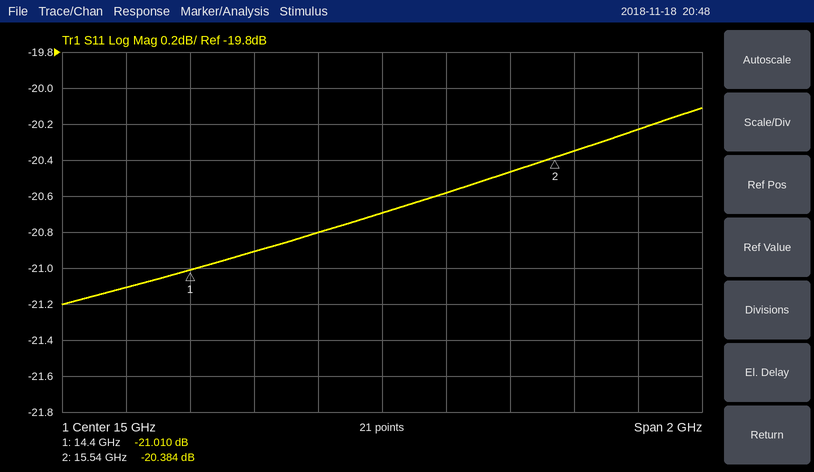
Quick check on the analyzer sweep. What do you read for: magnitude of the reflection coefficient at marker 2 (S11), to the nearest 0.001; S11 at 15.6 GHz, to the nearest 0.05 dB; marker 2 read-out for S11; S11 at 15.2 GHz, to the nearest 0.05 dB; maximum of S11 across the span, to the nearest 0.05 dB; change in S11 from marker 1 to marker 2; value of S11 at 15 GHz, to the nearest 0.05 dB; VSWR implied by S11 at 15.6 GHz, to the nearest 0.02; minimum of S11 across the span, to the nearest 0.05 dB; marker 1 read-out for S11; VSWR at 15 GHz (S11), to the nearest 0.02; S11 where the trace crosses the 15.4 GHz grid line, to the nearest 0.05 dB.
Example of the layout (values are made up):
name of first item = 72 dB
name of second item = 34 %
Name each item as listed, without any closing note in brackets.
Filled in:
magnitude of the reflection coefficient at marker 2 (S11), to the nearest 0.001 = 0.096
S11 at 15.6 GHz, to the nearest 0.05 dB = -20.35 dB
marker 2 read-out for S11 = -20.384 dB
S11 at 15.2 GHz, to the nearest 0.05 dB = -20.60 dB
maximum of S11 across the span, to the nearest 0.05 dB = -20.10 dB
change in S11 from marker 1 to marker 2 = 0.626 dB
value of S11 at 15 GHz, to the nearest 0.05 dB = -20.70 dB
VSWR implied by S11 at 15.6 GHz, to the nearest 0.02 = 1.22
minimum of S11 across the span, to the nearest 0.05 dB = -21.20 dB
marker 1 read-out for S11 = -21.010 dB
VSWR at 15 GHz (S11), to the nearest 0.02 = 1.20
S11 where the trace crosses the 15.4 GHz grid line, to the nearest 0.05 dB = -20.45 dB
